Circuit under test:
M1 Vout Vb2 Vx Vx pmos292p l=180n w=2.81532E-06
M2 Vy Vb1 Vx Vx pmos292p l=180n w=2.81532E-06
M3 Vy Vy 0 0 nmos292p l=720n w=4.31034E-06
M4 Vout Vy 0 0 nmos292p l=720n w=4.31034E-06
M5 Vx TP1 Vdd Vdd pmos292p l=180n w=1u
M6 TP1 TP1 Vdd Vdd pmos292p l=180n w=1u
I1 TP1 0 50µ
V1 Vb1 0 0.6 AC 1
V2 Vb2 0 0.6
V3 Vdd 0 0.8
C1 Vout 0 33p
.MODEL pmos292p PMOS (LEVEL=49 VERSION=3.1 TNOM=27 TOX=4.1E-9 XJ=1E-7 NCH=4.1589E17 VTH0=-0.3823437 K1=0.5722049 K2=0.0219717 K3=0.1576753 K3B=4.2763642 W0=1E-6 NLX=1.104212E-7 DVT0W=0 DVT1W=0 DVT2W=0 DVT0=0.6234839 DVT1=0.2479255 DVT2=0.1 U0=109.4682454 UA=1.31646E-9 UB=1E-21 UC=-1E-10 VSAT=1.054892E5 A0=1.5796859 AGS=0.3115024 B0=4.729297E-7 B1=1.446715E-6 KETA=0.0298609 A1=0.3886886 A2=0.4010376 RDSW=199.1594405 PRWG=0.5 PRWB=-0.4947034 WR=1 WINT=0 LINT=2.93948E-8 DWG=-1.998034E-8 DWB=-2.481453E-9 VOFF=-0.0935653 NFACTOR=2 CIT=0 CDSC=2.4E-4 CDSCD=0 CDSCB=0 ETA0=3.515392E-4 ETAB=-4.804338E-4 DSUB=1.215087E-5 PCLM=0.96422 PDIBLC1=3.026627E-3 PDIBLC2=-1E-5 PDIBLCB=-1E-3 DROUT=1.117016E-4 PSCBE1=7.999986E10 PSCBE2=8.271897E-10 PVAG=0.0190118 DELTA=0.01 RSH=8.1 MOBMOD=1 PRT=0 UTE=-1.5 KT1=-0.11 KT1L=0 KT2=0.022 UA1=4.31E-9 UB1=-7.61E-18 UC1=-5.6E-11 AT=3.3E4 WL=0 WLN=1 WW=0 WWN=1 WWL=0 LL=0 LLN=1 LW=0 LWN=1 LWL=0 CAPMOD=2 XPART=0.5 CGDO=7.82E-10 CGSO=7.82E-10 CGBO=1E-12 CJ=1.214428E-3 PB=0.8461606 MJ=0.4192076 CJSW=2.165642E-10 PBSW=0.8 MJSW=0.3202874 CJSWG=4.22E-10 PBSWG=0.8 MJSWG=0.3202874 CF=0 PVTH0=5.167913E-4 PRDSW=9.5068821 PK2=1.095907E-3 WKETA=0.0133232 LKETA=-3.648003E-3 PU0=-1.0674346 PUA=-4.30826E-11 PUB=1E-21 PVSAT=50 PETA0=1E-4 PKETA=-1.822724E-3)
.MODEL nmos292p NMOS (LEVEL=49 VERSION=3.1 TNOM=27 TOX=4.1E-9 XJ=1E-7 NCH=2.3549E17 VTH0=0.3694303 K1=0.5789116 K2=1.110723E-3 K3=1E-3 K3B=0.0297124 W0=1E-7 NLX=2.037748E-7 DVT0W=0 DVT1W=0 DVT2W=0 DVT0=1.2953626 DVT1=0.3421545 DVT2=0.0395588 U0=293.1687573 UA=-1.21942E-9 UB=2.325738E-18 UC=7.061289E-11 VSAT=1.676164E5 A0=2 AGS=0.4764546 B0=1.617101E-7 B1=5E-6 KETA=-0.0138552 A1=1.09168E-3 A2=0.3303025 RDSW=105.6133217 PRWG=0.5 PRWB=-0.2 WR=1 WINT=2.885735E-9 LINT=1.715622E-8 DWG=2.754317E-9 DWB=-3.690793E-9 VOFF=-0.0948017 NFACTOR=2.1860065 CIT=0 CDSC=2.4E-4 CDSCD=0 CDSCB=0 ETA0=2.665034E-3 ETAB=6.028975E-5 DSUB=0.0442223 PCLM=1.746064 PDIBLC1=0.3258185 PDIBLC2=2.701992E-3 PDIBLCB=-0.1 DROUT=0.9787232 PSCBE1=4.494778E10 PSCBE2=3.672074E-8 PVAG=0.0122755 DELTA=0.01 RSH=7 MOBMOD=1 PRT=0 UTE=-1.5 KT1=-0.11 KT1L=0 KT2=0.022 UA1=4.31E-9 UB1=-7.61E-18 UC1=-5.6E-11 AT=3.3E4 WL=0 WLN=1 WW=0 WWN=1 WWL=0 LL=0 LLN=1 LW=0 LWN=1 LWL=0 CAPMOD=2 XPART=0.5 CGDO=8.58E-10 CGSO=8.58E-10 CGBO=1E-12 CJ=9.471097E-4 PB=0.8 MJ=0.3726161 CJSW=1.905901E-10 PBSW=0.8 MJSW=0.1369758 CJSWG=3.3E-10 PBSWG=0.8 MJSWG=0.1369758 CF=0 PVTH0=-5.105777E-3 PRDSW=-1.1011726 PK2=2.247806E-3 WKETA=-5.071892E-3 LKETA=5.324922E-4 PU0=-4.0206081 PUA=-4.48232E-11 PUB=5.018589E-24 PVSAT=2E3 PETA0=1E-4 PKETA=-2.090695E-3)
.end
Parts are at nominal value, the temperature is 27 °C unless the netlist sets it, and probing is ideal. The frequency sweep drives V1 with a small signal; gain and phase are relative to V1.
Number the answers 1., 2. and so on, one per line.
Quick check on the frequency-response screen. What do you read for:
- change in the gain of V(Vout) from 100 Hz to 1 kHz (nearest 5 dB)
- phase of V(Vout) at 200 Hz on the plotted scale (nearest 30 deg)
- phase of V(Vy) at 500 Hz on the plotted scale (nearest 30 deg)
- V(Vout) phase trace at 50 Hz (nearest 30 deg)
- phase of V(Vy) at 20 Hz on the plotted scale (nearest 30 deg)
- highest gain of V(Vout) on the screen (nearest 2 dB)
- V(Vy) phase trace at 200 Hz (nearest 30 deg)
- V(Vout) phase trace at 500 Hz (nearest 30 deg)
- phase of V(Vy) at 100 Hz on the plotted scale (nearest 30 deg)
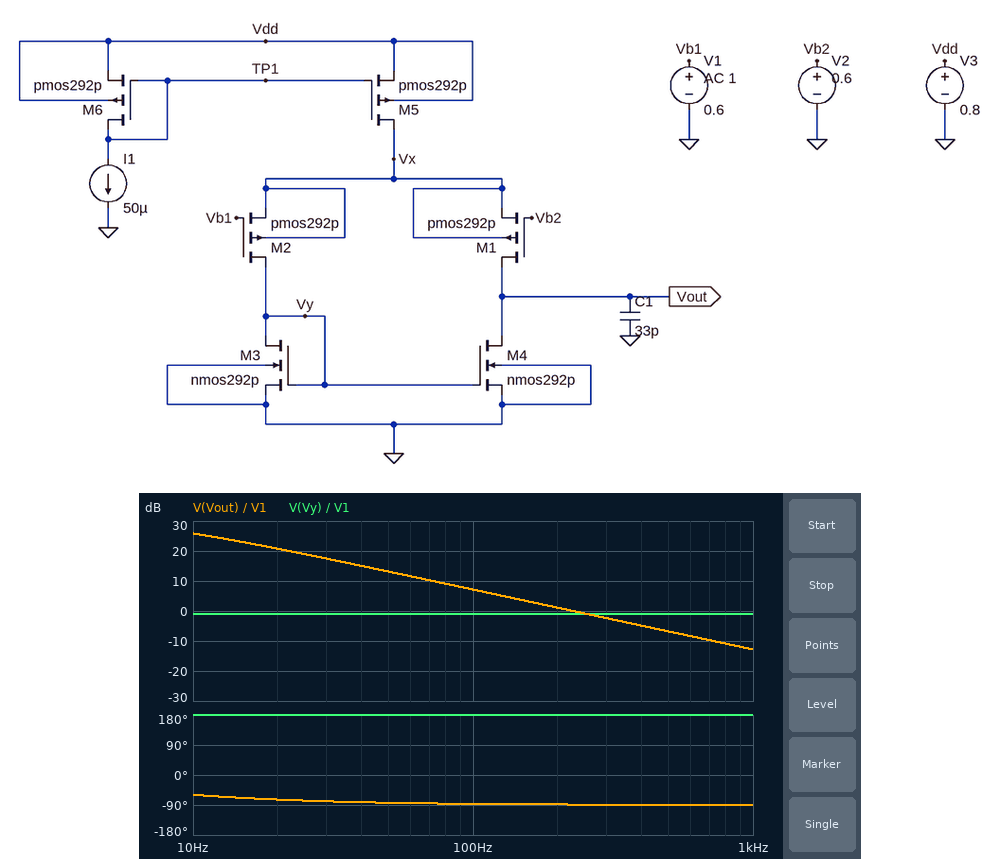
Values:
1. -20 dB
2. -90 deg
3. 180 deg
4. -90 deg
5. 180 deg
6. 26 dB
7. 180 deg
8. -90 deg
9. 180 deg
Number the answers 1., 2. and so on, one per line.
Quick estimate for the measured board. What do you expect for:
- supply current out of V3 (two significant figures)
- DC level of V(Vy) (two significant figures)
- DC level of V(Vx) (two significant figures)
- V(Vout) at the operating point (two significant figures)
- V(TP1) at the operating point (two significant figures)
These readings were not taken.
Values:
1. 50 µA
2. 190 mV
3. 800 mV
4. 190 mV
5. -150 mV
